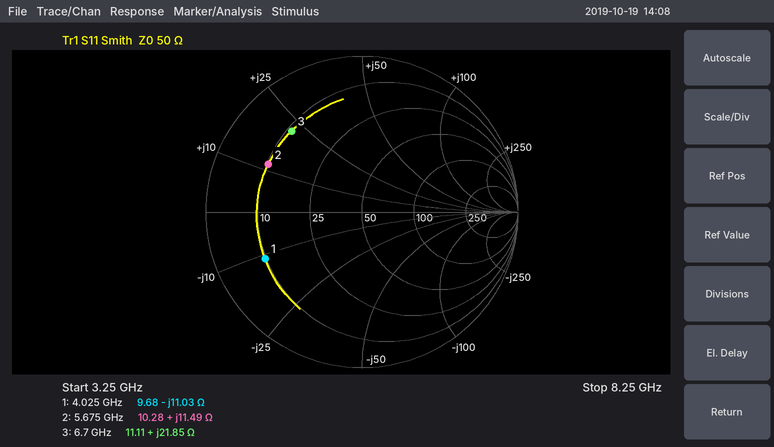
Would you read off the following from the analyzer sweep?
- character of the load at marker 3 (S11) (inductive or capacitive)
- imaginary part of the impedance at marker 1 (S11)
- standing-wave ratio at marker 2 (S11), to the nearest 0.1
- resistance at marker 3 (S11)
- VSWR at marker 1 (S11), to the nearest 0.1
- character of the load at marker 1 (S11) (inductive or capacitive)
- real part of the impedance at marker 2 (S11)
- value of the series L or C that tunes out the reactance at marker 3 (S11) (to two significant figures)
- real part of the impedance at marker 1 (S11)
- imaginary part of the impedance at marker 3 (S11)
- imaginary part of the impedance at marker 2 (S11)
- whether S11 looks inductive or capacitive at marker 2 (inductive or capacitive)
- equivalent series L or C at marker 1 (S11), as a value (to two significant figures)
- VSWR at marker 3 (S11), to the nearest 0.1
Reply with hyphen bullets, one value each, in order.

- inductive
- -11.03 Ω
- 5.1
- 11.11 Ω
- 5.4
- capacitive
- 10.28 Ω
- 1.1 pF
- 9.68 Ω
- +21.85 Ω
- +11.49 Ω
- inductive
- 3.6 pF
- 5.4
